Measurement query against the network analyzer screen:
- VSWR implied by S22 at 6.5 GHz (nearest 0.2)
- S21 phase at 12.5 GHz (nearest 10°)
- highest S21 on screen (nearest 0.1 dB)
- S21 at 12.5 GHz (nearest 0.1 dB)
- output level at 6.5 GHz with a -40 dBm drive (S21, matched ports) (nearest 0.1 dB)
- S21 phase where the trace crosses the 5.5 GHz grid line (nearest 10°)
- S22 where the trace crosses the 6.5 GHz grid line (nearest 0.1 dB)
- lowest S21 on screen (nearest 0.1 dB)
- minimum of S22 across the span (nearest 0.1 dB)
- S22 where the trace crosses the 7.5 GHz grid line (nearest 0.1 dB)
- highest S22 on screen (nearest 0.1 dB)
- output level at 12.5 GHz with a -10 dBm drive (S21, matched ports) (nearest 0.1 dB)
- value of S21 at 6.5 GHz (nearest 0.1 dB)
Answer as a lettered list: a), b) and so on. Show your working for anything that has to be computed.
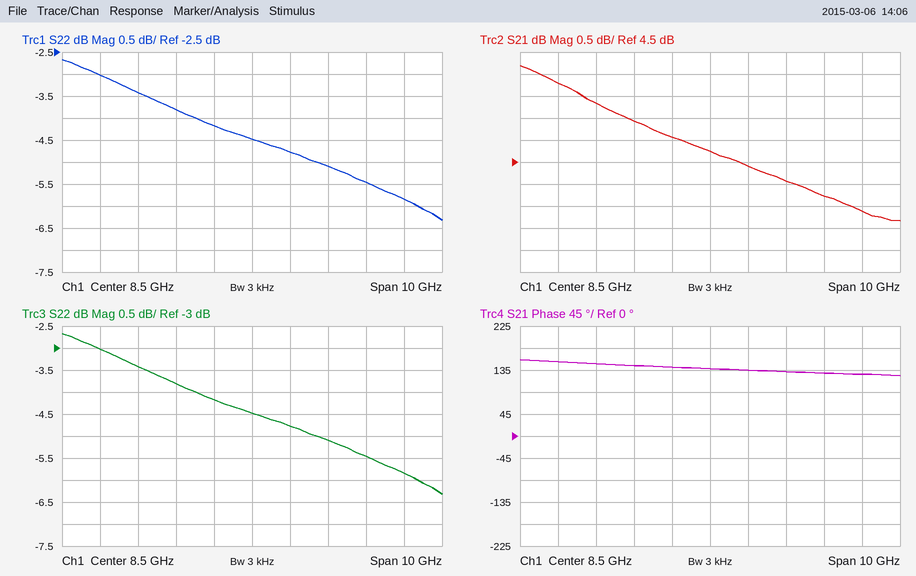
a) |Γ| = 10^(-3.8/20) = 0.6457; VSWR = (1 + 0.6457)/(1 − 0.6457) ≈ 4.6
b) 130°
c) 6.7 dB
d) 3.4 dB
e) -40 dBm + (5.4 dB) = -34.6 dBm
f) 150°
g) -3.8 dB
h) 3.2 dB
i) -6.3 dB
j) -4.2 dB
k) -2.7 dB
l) -10 dBm + (3.4 dB) = -6.6 dBm
m) 5.4 dB
